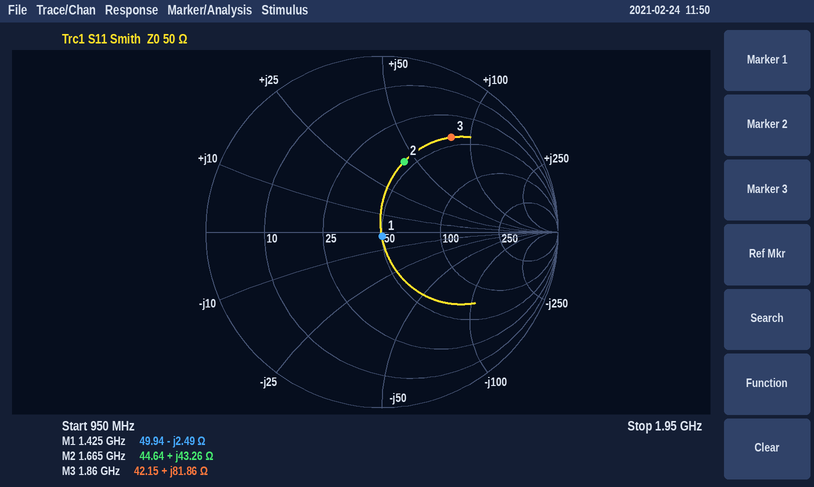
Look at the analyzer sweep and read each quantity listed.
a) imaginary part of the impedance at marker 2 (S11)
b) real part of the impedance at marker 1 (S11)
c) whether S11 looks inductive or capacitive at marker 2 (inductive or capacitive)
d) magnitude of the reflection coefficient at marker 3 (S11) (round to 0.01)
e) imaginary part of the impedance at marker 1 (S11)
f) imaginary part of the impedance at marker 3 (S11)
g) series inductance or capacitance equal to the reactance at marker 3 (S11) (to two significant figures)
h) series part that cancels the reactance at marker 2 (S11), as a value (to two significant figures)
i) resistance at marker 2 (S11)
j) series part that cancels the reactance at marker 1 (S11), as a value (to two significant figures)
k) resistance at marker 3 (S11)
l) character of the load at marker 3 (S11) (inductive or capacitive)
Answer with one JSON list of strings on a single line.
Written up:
["+43.26 Ω", "49.94 Ω", "inductive", "0.67", "-2.49 Ω", "+81.86 Ω", "7.0 nH", "2.2 pF", "44.64 Ω", "280 pH", "42.15 Ω", "inductive"]
